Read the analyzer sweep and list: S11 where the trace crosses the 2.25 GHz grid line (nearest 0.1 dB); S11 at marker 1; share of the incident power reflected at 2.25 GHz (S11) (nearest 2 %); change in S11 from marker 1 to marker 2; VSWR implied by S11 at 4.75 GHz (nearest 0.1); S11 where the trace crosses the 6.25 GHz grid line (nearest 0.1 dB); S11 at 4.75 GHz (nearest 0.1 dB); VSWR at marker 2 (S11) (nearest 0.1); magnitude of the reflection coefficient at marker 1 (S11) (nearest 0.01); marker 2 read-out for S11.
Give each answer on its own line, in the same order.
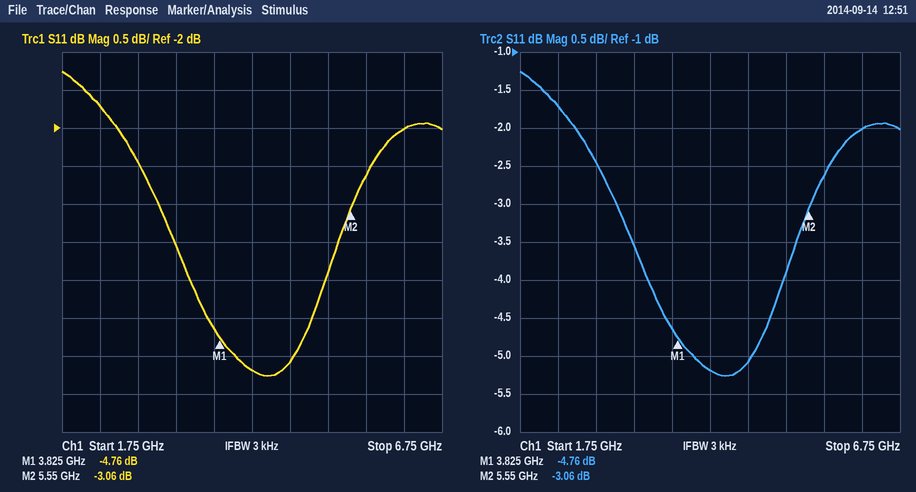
-1.7 dB
-4.76 dB
68 %
1.70 dB
3.5
-2.0 dB
-5.1 dB
5.7
0.58
-3.06 dB
